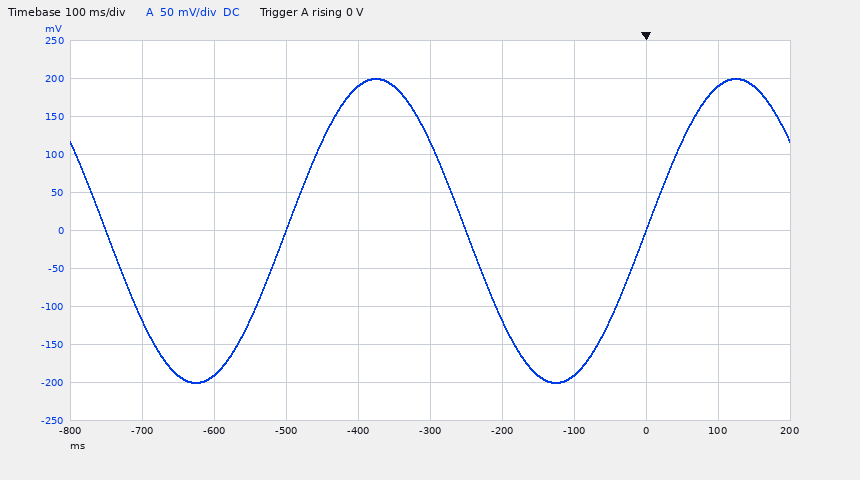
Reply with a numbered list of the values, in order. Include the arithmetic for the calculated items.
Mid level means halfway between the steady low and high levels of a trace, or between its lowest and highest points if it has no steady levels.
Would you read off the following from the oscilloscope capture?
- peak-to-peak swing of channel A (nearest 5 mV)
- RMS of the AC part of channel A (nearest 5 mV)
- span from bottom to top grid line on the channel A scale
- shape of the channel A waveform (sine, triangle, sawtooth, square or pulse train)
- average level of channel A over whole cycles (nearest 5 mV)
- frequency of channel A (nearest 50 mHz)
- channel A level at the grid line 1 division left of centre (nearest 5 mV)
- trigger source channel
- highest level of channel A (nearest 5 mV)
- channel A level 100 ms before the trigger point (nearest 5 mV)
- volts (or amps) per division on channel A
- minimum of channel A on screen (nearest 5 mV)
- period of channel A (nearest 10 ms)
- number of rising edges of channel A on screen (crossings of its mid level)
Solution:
1. 200 mV − (-200 mV) = 400 mV
2. 400 mV / (2√2) ≈ 141 mV, so 140 mV to the nearest 5 mV
3. 500 mV
4. sine
5. (200 mV + (-200 mV)) / 2 ≈ 0 mV
6. 1 / 500 ms ≈ 2.00 Hz
7. 190 mV
8. channel A
9. 200 mV
10. -190 mV
11. 50 mV
12. -200 mV
13. 500 ms
14. 2
